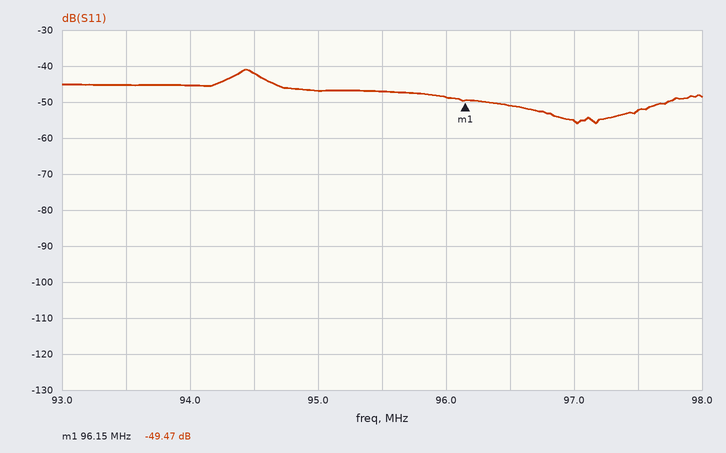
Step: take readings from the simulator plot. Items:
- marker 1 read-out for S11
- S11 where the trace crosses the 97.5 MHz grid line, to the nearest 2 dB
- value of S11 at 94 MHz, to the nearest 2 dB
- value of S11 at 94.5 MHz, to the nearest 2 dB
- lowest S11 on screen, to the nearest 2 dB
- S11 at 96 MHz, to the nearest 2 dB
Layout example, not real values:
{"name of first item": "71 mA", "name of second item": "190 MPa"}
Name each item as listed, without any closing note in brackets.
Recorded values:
{"marker 1 read-out for S11": "-49.47 dB", "S11 where the trace crosses the 97.5 MHz grid line, to the nearest 2 dB": "-52 dB", "value of S11 at 94 MHz, to the nearest 2 dB": "-46 dB", "value of S11 at 94.5 MHz, to the nearest 2 dB": "-42 dB", "lowest S11 on screen, to the nearest 2 dB": "-56 dB", "S11 at 96 MHz, to the nearest 2 dB": "-48 dB"}
